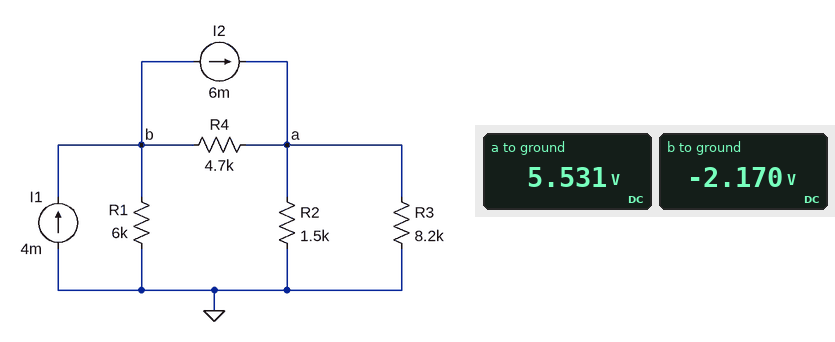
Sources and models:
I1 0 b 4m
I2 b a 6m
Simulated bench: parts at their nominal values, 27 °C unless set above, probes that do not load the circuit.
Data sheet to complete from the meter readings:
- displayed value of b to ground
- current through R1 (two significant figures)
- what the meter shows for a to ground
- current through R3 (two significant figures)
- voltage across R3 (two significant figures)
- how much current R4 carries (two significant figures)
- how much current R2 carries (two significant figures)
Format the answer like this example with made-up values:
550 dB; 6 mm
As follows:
-2.170 V; 360 µA; 5.531 V; 670 µA; 5.5 V; 1.6 mA; 3.7 mA
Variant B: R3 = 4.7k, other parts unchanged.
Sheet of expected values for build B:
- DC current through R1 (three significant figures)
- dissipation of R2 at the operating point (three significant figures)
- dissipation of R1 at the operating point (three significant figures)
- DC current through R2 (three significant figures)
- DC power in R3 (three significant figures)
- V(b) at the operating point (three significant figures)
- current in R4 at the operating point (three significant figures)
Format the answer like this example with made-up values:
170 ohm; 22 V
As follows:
410 µA; 16.8 mW; 1.01 mW; 3.34 mA; 5.35 mW; -2.46 V; 1.59 mA
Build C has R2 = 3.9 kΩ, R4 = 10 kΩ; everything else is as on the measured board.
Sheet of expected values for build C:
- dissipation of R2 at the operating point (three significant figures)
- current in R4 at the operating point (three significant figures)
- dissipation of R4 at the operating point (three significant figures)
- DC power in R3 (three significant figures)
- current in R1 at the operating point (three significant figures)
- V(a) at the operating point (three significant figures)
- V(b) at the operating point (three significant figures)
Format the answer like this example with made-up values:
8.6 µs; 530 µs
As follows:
36.4 mW; 1.49 mA; 22.3 mW; 17.3 mW; 506 µA; 11.9 V; -3.03 V
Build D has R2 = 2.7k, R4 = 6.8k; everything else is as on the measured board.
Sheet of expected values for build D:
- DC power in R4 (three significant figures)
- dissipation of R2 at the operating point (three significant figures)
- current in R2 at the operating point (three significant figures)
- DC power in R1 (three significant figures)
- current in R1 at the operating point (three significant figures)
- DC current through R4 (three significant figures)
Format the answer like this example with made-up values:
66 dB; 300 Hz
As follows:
18.1 mW; 29.2 mW; 3.29 mA; 818 µW; 369 µA; 1.63 mA
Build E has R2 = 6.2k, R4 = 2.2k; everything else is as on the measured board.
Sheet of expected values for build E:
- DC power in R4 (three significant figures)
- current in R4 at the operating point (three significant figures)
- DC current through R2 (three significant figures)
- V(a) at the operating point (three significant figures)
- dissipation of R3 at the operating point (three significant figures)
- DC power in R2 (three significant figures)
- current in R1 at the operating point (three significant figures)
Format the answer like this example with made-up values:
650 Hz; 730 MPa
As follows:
17.6 mW; 2.83 mA; 1.81 mA; 11.2 V; 15.3 mW; 20.2 mW; 829 µA
